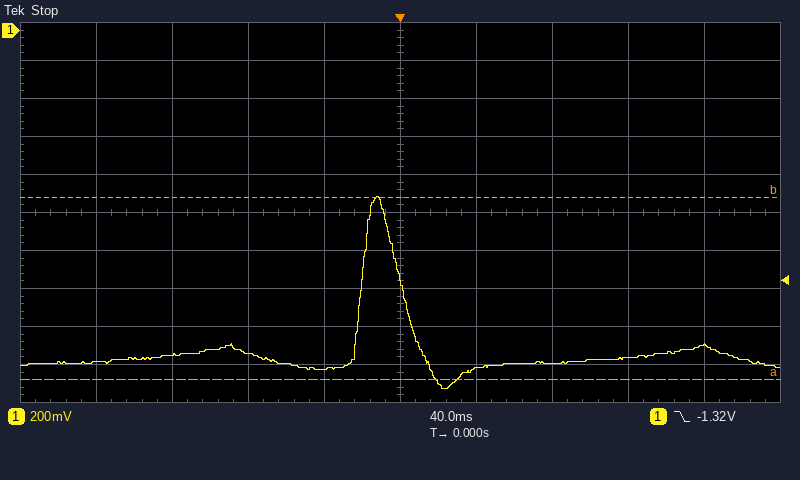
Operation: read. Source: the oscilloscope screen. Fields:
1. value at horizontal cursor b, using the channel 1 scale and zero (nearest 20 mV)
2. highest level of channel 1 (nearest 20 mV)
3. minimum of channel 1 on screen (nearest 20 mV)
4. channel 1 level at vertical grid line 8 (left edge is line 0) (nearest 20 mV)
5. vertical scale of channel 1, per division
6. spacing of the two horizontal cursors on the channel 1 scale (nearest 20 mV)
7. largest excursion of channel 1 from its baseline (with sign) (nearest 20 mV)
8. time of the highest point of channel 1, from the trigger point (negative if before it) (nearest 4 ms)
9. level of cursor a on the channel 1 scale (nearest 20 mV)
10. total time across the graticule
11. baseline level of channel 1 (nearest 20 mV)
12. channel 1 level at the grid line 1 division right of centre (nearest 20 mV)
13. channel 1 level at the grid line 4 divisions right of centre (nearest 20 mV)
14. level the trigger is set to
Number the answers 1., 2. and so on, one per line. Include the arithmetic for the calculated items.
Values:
1. -880 mV
2. -880 mV
3. -1.88 V
4. -1.72 V
5. 200 mV
6. 960 mV
7. -880 mV − (-1.74 V) = +860 mV
8. -12 ms
9. -1.84 V
10. 400 ms
11. -1.74 V
12. -1.78 V
13. -1.66 V
14. -1.32 V
